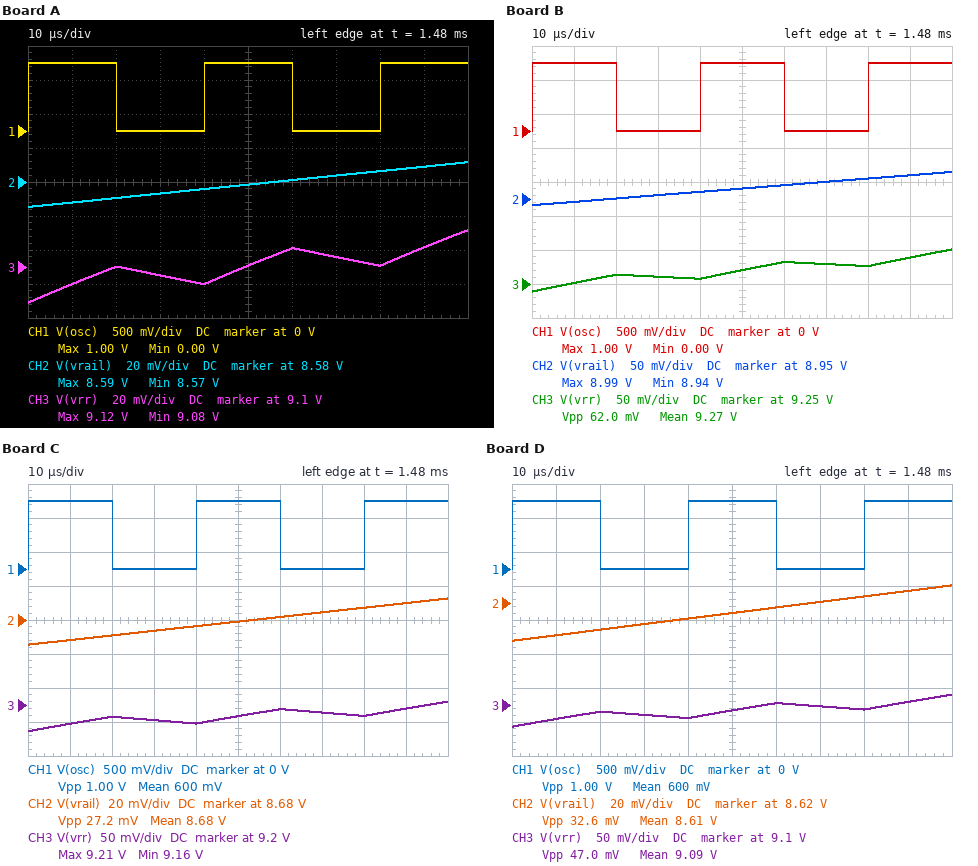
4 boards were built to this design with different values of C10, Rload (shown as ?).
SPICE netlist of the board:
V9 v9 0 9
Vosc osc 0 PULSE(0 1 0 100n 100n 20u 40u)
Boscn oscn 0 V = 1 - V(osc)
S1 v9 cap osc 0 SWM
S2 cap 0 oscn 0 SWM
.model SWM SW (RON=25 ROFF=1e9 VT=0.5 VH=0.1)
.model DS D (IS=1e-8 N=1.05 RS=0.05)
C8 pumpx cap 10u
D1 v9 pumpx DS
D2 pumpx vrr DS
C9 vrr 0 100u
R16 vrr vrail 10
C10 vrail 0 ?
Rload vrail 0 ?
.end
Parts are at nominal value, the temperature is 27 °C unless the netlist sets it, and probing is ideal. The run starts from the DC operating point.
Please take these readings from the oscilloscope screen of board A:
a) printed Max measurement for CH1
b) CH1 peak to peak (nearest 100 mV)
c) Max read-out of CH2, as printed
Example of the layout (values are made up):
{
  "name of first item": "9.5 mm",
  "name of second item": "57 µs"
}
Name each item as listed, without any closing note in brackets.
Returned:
{
  "printed Max measurement for CH1": "1.00 V",
  "CH1 peak to peak": "1.0 V",
  "Max read-out of CH2, as printed": "8.59 V"
}
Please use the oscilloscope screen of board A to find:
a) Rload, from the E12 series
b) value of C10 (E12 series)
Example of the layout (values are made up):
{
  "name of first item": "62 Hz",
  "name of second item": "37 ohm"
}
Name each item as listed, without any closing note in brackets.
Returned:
{
  "Rload, from the E12 series": "1.8 kΩ",
  "value of C10": "180 µF"
}
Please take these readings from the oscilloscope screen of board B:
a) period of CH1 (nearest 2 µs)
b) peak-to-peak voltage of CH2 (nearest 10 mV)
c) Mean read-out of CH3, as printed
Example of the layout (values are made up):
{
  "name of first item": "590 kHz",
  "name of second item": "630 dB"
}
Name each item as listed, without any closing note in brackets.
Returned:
{
  "period of CH1": "40 µs",
  "peak-to-peak voltage of CH2": "50 mV",
  "Mean read-out of CH3, as printed": "9.27 V"
}
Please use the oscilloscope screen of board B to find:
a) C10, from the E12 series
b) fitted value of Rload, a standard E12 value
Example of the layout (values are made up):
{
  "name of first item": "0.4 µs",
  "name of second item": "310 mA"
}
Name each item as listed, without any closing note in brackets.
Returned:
{
  "C10, from the E12 series": "47 µF",
  "fitted value of Rload, a standard E12 value": "1.2 kΩ"
}
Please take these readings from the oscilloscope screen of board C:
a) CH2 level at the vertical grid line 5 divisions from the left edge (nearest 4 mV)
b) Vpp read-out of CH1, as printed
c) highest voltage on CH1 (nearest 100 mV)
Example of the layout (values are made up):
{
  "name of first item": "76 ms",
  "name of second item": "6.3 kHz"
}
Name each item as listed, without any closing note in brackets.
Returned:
{
  "CH2 level at the vertical grid line 5 divisions from the left edge": "8.680 V",
  "Vpp read-out of CH1, as printed": "1.00 V",
  "highest voltage on CH1": "1.0 V"
}
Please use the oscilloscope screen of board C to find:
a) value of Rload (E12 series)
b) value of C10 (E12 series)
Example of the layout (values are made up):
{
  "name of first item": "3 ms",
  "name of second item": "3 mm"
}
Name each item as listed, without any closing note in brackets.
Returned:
{
  "value of Rload": "5.6 kΩ",
  "value of C10": "180 µF"
}
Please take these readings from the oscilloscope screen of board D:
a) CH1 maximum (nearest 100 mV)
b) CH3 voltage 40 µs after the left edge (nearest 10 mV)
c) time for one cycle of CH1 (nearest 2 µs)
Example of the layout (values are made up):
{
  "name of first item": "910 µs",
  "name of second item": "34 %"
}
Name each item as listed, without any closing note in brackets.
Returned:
{
  "CH1 maximum": "1.0 V",
  "CH3 voltage 40 µs after the left edge": "9.08 V",
  "time for one cycle of CH1": "40 µs"
}
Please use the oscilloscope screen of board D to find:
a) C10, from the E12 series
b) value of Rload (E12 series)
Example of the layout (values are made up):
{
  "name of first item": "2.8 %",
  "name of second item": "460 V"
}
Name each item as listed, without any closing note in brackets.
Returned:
{
  "C10, from the E12 series": "120 µF",
  "value of Rload": "1 kΩ"
}
